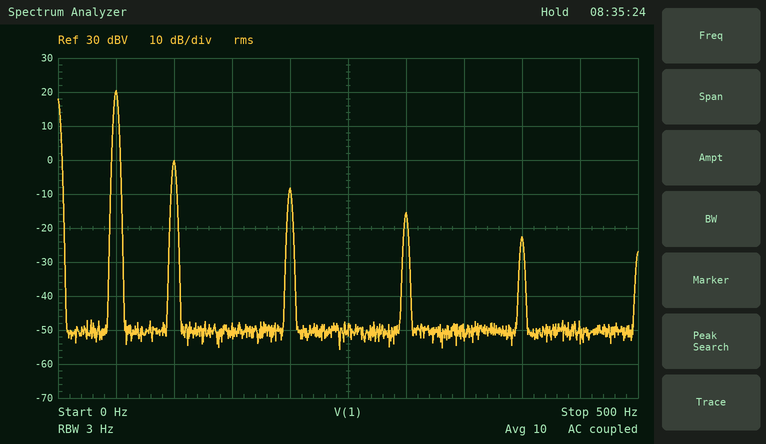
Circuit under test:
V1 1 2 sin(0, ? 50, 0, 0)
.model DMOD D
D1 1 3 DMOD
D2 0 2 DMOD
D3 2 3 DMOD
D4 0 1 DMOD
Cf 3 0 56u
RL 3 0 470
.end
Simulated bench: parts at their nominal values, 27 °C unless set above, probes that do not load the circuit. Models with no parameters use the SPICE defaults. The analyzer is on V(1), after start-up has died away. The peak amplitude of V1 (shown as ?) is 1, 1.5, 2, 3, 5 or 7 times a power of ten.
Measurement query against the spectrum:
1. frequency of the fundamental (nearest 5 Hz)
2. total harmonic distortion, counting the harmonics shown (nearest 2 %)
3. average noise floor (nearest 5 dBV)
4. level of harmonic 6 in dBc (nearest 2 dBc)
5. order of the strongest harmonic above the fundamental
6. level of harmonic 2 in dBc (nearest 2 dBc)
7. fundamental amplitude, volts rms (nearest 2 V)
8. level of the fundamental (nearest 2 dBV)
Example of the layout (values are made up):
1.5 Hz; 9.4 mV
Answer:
50 Hz; 10 %; -50 dBV; -36 dBc; 2; -20 dBc; 10 V; 20 dBV
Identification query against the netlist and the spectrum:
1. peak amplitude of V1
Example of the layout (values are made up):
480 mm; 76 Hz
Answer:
30 V
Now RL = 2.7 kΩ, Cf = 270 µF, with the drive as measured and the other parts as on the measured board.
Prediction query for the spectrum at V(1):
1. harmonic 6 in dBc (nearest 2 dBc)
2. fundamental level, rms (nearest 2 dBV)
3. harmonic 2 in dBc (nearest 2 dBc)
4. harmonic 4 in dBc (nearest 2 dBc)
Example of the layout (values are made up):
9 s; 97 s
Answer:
-58 dBc; 20 dBV; -48 dBc; -54 dBc
